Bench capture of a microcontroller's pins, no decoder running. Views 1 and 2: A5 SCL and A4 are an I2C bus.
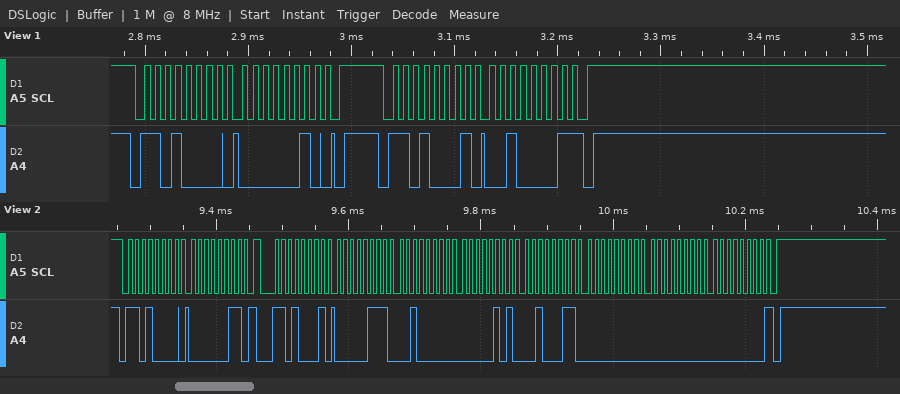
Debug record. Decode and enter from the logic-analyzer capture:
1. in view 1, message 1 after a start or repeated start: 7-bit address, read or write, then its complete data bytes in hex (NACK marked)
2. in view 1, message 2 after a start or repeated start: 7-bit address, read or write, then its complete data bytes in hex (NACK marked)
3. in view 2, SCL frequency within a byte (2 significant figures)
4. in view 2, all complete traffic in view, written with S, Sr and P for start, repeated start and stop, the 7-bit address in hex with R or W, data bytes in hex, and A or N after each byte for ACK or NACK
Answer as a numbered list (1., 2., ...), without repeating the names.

1. 0x68 write: 02
2. 0x68 read: 21 NACK
3. 100 kHz
4. S 68W A 03 A Sr 68R A 07 A 20 A 05 A 23 A 00 A 00 A 00 N P
